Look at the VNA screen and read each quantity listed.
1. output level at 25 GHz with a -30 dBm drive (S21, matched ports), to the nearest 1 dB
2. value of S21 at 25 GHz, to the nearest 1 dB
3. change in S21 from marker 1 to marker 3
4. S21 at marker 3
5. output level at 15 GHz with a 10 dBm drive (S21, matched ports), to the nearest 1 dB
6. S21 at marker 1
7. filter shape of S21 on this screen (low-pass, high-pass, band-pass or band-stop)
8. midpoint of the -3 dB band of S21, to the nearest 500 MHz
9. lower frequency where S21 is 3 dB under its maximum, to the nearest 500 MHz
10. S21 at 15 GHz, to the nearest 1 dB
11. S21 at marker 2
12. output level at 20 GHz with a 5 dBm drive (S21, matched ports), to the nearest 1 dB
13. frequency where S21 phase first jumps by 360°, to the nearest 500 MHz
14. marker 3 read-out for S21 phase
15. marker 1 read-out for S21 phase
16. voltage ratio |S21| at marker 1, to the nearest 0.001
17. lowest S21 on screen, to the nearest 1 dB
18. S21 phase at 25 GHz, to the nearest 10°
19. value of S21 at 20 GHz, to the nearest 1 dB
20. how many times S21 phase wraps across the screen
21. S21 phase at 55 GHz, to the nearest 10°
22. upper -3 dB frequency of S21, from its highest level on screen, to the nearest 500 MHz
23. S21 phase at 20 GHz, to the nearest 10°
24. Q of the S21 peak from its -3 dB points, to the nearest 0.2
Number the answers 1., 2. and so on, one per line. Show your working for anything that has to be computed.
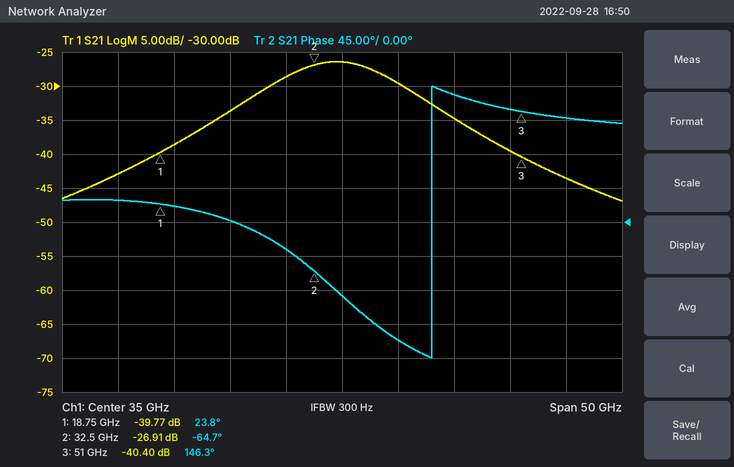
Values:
1. -30 dBm + (-34 dB) = -64 dBm
2. -34 dB
3. -40.4 − (-39.77) = -0.63 dB
4. -40.40 dB
5. 10 dBm + (-43 dB) = -33 dBm
6. -39.77 dB
7. band-pass
8. 34.5 GHz
9. 29.0 GHz
10. -43 dB
11. -26.91 dB
12. 5 dBm + (-39 dB) = -34 dBm
13. 43.0 GHz
14. 146.3°
15. 23.8°
16. 10^(-39.77/20) ≈ 0.010
17. -47 dB
18. 0°
19. -39 dB
20. 1
21. 140°
22. 40.0 GHz
23. 20°
24. 34.5 GHz / 11 GHz ≈ 3.14, so 3.2 to the nearest 0.2
